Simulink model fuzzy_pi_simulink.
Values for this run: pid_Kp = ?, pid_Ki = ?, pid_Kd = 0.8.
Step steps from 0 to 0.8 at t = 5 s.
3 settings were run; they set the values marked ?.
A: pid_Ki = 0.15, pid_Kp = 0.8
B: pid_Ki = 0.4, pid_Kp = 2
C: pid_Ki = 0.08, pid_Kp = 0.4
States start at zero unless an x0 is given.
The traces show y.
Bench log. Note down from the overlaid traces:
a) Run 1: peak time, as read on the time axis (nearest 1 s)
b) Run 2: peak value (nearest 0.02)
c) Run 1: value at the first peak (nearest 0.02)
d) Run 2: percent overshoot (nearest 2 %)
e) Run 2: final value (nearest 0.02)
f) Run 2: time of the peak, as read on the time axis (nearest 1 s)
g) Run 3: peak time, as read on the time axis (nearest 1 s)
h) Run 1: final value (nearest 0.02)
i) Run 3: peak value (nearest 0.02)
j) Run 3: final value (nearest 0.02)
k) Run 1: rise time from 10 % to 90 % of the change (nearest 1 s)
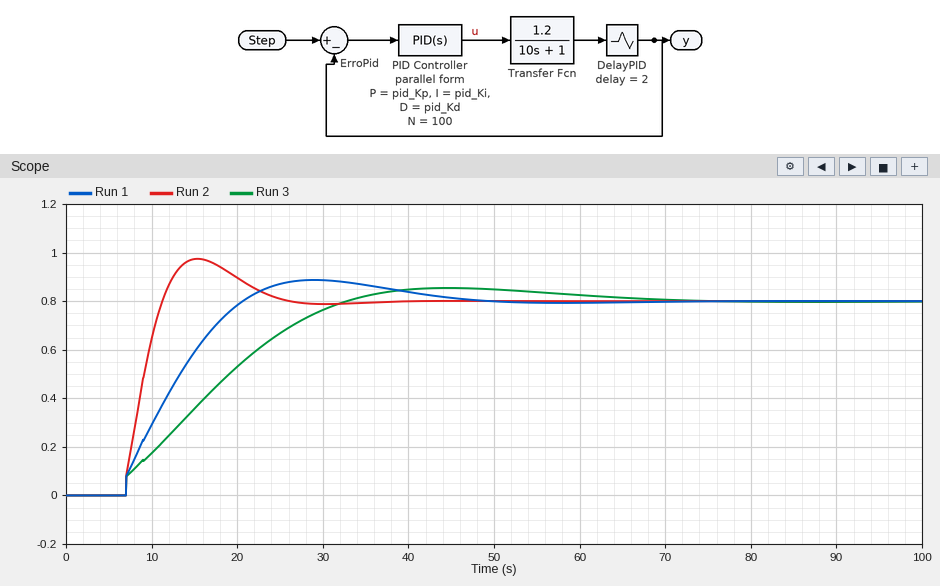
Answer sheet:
29 s
0.98
0.88
22 %
0.80
15 s
45 s
0.80
0.86
0.80
11 s
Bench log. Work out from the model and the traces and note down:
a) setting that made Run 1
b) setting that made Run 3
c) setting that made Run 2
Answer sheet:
A
C
B
